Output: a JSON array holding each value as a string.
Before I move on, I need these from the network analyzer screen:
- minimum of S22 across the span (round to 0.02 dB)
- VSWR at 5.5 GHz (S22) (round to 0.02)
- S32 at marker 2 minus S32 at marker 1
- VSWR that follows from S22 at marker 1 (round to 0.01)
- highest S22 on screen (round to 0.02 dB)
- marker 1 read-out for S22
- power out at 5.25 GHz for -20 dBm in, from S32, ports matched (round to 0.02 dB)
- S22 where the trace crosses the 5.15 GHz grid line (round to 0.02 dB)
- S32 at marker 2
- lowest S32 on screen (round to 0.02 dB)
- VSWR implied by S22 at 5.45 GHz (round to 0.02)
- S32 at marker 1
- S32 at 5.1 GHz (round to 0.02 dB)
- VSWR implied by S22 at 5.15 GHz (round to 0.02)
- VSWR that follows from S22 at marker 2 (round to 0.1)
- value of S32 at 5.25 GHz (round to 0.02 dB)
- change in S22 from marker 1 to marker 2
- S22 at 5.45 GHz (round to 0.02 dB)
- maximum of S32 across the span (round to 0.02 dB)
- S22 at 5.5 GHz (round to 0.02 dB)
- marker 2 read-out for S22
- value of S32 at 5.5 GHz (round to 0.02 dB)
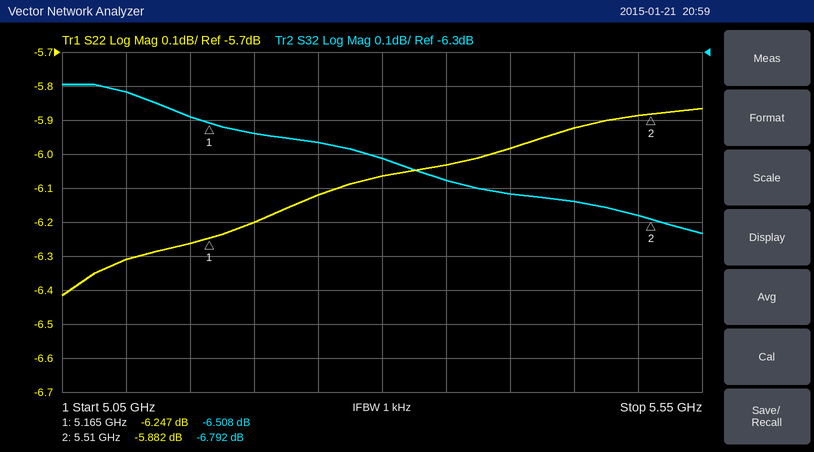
["-6.42 dB", "3.06", "-0.284 dB", "2.90", "-5.86 dB", "-6.247 dB", "-26.56 dBm", "-6.26 dB", "-6.792 dB", "-6.84 dB", "3.04", "-6.508 dB", "-6.42 dB", "2.90", "3.1", "-6.56 dB", "0.365 dB", "-5.92 dB", "-6.40 dB", "-5.88 dB", "-5.882 dB", "-6.78 dB"]
